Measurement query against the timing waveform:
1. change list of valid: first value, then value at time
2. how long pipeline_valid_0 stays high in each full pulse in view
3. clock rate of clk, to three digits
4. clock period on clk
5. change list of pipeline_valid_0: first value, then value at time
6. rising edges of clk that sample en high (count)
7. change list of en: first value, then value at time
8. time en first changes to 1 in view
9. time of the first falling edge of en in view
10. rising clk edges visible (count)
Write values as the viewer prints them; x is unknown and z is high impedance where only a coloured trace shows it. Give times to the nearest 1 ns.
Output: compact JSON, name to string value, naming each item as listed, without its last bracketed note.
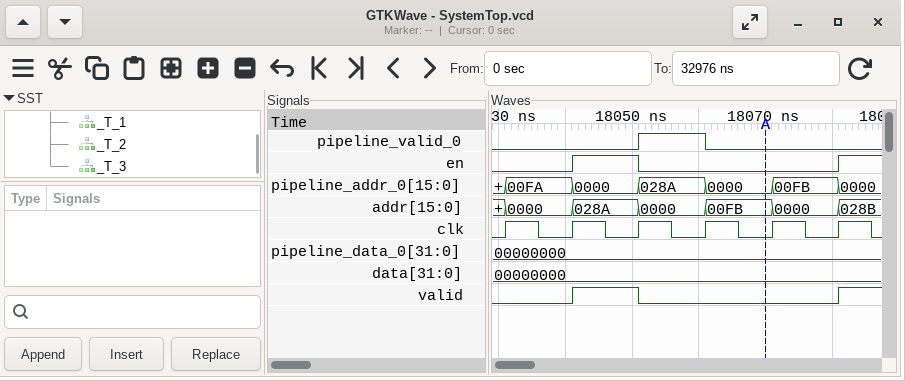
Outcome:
{"change list of valid: first value, then value at time": "0, 1 at 18041 ns, 0 at 18051 ns, 1 at 18081 ns", "how long pipeline_valid_0 stays high in each full pulse in view": "10 ns", "clock rate of clk, to three digits": "100 MHz", "clock period on clk": "10 ns", "change list of pipeline_valid_0: first value, then value at time": "0, 1 at 18051 ns, 0 at 18061 ns", "rising edges of clk that sample en high": "1", "change list of en: first value, then value at time": "0, 1 at 18041 ns, 0 at 18051 ns, 1 at 18081 ns", "time en first changes to 1 in view": "18041 ns", "time of the first falling edge of en in view": "18051 ns", "rising clk edges visible": "6"}
